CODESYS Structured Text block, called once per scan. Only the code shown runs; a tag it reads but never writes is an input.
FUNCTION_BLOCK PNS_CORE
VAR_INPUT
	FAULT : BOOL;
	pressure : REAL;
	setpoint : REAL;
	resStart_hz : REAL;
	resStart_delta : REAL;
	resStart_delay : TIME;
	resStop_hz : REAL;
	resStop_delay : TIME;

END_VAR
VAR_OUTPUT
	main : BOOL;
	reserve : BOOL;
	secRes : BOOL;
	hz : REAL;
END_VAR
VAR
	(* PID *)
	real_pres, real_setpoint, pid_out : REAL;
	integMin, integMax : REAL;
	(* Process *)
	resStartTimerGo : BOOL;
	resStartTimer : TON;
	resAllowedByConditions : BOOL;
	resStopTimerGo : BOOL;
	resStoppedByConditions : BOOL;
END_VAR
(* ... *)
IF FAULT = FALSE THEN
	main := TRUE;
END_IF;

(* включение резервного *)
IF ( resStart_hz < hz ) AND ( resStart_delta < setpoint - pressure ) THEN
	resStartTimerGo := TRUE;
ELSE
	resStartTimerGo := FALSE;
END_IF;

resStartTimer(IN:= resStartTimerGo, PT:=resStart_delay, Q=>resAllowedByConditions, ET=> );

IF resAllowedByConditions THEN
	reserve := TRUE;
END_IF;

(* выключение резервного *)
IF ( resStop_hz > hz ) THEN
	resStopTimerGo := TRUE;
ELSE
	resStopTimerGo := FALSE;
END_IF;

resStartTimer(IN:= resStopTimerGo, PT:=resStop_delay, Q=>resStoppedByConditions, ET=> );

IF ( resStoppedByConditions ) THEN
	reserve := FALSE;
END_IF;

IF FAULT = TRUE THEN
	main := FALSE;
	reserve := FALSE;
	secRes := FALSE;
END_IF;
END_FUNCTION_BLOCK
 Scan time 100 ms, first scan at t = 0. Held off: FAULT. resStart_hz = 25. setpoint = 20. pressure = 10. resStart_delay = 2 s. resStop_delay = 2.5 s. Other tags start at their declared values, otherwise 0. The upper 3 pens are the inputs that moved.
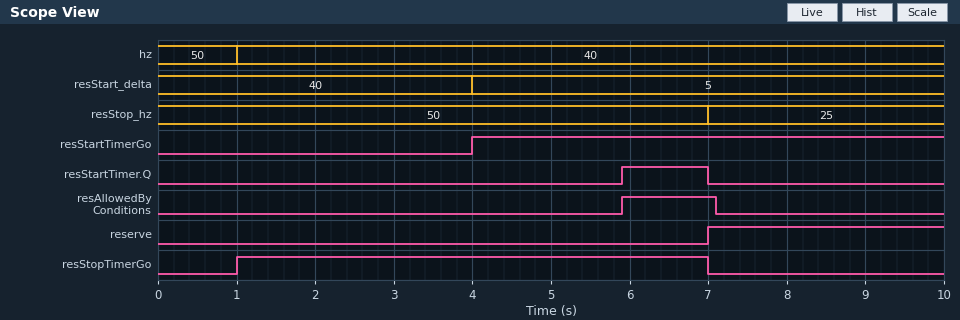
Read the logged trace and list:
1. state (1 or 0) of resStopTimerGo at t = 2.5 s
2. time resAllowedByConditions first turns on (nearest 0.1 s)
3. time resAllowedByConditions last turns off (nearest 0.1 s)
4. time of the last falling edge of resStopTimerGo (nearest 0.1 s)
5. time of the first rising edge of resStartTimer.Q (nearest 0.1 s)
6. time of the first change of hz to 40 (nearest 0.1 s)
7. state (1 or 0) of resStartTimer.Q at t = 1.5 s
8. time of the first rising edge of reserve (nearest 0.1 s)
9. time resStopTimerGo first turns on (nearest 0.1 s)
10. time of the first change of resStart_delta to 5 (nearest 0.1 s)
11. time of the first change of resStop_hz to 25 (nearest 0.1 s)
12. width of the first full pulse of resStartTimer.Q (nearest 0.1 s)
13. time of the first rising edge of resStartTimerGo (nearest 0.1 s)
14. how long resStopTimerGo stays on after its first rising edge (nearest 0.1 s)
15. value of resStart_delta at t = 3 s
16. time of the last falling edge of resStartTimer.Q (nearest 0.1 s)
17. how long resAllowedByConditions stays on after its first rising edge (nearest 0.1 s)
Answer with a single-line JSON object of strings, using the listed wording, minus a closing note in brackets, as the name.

{"state (1 or 0) of resStopTimerGo at t = 2.5 s": "1", "time resAllowedByConditions first turns on": "5.9 s", "time resAllowedByConditions last turns off": "7.1 s", "time of the last falling edge of resStopTimerGo": "7.0 s", "time of the first rising edge of resStartTimer.Q": "5.9 s", "time of the first change of hz to 40": "1.0 s", "state (1 or 0) of resStartTimer.Q at t = 1.5 s": "0", "time of the first rising edge of reserve": "7.0 s", "time resStopTimerGo first turns on": "1.0 s", "time of the first change of resStart_delta to 5": "4.0 s", "time of the first change of resStop_hz to 25": "7.0 s", "width of the first full pulse of resStartTimer.Q": "1.1 s", "time of the first rising edge of resStartTimerGo": "4.0 s", "how long resStopTimerGo stays on after its first rising edge": "6.0 s", "value of resStart_delta at t = 3 s": "40", "time of the last falling edge of resStartTimer.Q": "7.0 s", "how long resAllowedByConditions stays on after its first rising edge": "1.2 s"}
